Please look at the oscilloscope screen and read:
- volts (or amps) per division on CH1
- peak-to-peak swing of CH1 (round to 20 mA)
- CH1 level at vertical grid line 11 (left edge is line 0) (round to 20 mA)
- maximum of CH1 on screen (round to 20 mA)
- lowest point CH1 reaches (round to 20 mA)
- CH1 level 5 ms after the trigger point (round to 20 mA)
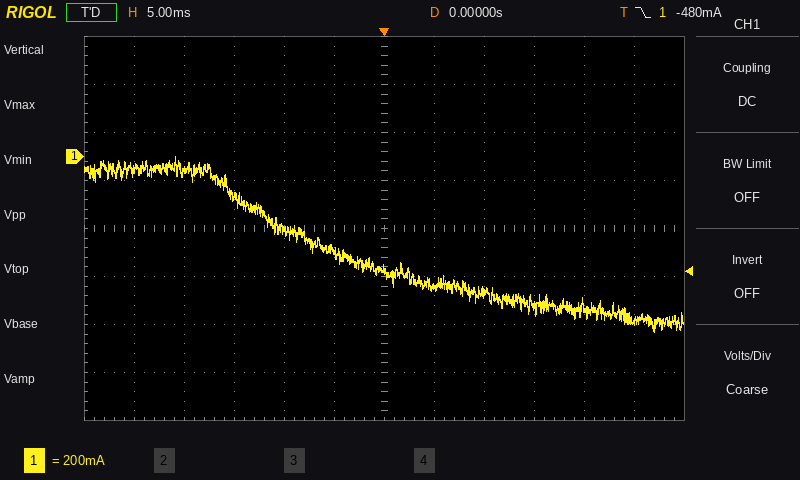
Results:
200 mA
720 mA
-680 mA
0 mA
-720 mA
-540 mA
